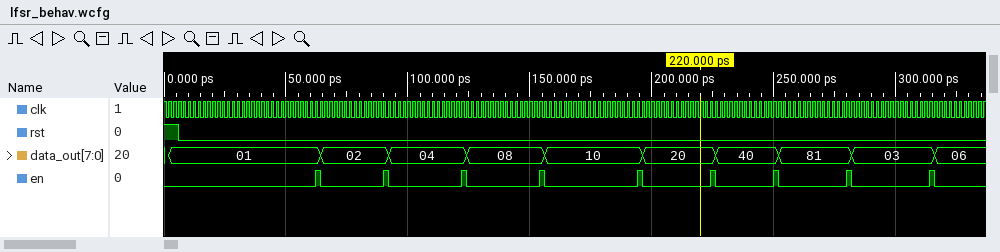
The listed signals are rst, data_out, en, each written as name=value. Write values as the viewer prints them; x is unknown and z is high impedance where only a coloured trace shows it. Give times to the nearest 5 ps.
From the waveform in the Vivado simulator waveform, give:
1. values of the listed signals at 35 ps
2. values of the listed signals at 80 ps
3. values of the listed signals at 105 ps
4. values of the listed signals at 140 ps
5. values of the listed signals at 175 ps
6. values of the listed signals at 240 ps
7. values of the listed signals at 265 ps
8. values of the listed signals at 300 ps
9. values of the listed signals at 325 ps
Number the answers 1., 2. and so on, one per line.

1. rst=0, data_out=01, en=0
2. rst=0, data_out=02, en=0
3. rst=0, data_out=04, en=0
4. rst=0, data_out=08, en=0
5. rst=0, data_out=10, en=0
6. rst=0, data_out=40, en=0
7. rst=0, data_out=81, en=0
8. rst=0, data_out=03, en=0
9. rst=0, data_out=06, en=0
